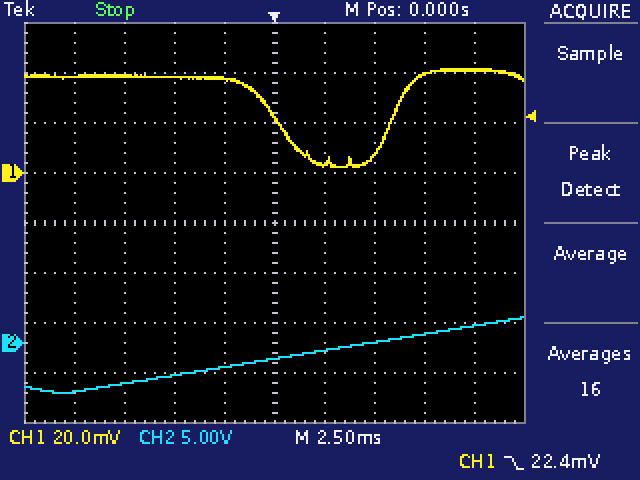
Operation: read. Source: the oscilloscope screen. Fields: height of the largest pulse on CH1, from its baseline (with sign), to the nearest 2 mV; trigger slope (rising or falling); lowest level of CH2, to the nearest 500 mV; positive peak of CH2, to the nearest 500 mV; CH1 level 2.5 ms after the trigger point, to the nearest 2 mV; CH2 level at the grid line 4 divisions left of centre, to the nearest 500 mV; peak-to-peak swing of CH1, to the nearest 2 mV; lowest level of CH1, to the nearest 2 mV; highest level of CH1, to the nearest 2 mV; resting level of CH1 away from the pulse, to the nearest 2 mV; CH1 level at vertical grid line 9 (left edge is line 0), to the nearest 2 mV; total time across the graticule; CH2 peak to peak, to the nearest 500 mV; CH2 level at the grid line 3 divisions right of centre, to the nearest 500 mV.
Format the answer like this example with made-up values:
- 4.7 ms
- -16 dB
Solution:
- -36 mV
- falling
- -5.0 V
- 2.5 V
- 4 mV
- -5.0 V
- 40 mV
- 2 mV
- 42 mV
- 38 mV
- 42 mV
- 25 ms
- 7.5 V
- 1.0 V
